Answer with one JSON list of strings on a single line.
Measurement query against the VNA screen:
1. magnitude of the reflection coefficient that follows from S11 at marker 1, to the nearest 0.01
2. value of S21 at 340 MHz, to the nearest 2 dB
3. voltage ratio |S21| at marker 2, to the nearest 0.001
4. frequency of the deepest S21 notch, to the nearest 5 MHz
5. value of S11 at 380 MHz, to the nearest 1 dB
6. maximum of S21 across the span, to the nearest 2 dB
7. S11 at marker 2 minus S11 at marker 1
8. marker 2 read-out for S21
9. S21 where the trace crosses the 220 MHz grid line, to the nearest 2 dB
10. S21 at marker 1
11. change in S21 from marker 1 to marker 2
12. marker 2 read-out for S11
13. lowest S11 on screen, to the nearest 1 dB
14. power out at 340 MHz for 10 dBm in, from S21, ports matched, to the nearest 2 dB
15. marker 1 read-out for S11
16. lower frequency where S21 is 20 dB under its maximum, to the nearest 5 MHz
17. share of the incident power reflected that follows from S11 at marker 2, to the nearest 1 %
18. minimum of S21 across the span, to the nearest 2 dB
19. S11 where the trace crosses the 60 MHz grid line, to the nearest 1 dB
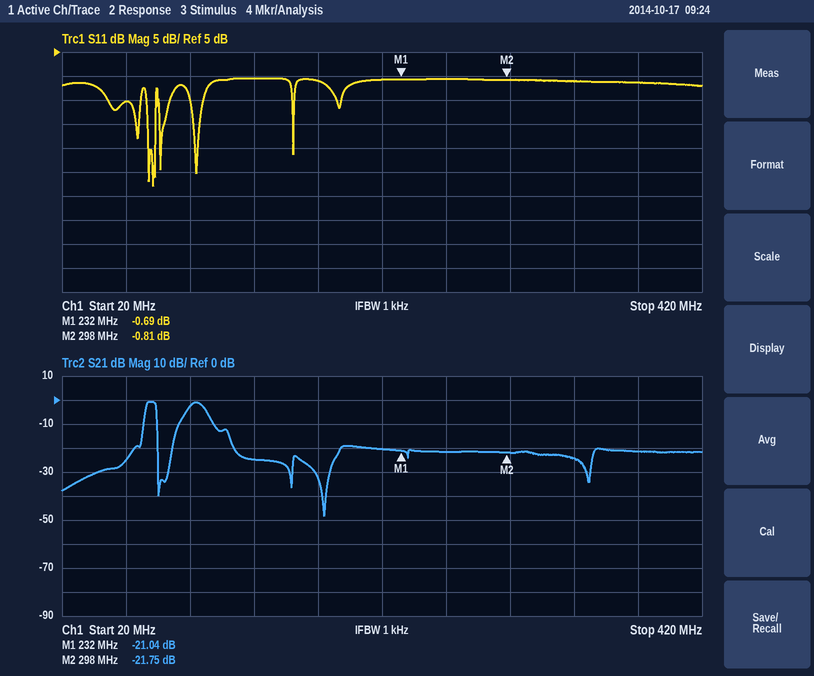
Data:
["0.92", "-24 dB", "0.082", "185 MHz", "-1 dB", "0 dB", "-0.12 dB", "-21.75 dB", "-20 dB", "-21.04 dB", "-0.71 dB", "-0.81 dB", "-23 dB", "-14 dBm", "-0.69 dB", "65 MHz", "83 %", "-48 dB", "-5 dB"]
